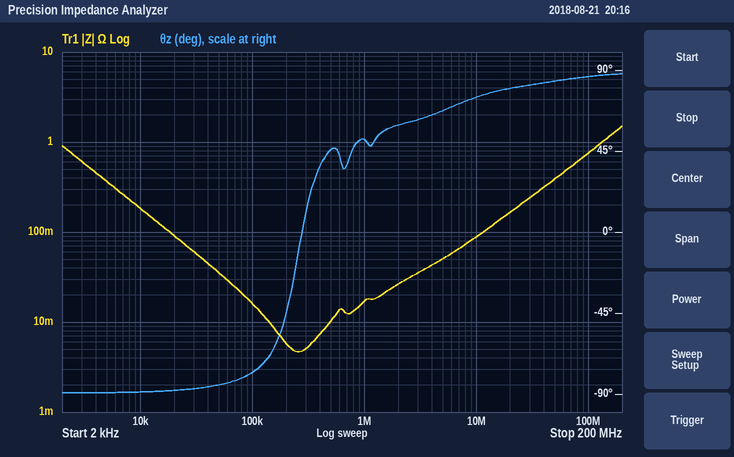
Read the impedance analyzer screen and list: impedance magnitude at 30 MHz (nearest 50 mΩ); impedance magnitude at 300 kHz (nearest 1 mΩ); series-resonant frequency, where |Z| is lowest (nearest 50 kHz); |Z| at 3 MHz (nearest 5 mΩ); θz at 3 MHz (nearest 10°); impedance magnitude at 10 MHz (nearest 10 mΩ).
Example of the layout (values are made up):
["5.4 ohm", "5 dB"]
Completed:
["250 mΩ", "5 mΩ", "250 kHz", "35 mΩ", "60°", "90 mΩ"]
